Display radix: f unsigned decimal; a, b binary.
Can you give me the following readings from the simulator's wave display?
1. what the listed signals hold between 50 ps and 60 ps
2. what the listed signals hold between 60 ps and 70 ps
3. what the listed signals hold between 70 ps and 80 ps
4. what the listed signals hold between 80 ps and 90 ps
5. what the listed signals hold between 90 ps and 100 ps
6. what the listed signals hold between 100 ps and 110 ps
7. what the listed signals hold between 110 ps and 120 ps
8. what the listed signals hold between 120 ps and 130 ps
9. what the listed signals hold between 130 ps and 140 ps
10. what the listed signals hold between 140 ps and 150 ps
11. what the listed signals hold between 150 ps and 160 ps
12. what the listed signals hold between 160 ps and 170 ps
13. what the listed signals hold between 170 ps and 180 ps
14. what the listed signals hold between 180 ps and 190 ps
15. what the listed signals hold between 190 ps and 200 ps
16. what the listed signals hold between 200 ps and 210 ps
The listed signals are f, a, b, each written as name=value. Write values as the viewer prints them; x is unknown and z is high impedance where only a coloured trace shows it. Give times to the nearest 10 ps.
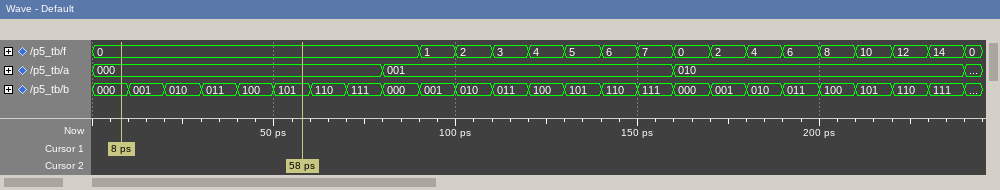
f=0, a=000, b=101
f=0, a=000, b=110
f=0, a=000, b=111
f=0, a=001, b=000
f=1, a=001, b=001
f=2, a=001, b=010
f=3, a=001, b=011
f=4, a=001, b=100
f=5, a=001, b=101
f=6, a=001, b=110
f=7, a=001, b=111
f=0, a=010, b=000
f=2, a=010, b=001
f=4, a=010, b=010
f=6, a=010, b=011
f=8, a=010, b=100
